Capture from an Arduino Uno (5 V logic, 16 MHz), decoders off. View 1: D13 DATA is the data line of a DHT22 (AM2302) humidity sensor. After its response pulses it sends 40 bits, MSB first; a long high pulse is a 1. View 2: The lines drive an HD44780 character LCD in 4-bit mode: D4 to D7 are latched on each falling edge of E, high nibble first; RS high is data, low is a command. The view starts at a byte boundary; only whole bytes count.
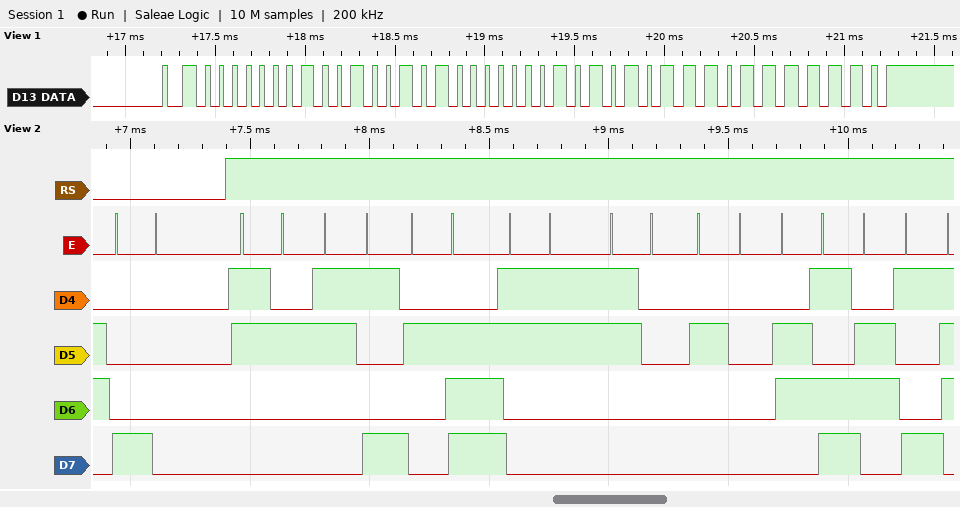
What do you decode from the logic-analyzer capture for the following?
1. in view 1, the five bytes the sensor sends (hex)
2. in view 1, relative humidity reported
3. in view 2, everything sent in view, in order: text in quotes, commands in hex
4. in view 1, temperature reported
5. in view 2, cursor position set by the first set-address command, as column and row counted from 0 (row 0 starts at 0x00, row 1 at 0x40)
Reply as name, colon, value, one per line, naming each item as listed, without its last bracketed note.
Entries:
in view 1, the five bytes the sensor sends: 01 25 01 57 7E
in view 1, relative humidity reported: 29.3 %
in view 2, everything sent in view, in order: text in quotes, commands in hex: 0x80 "29.30 mi"
in view 1, temperature reported: 34.3 °C
in view 2, cursor position set by the first set-address command, as column and row counted from 0: column 0, row 0
